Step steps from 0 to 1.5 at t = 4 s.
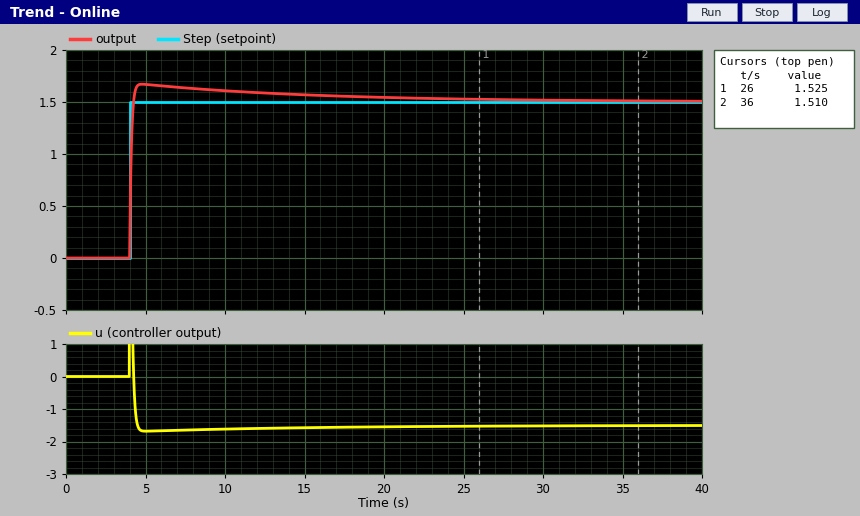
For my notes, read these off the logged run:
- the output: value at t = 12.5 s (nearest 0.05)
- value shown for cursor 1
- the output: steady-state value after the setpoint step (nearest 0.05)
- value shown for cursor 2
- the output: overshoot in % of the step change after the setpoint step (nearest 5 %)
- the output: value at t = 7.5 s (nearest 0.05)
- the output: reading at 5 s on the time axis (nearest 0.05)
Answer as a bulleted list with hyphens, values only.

- 1.60
- 1.525
- 1.50
- 1.510
- 10 %
- 1.65
- 1.65
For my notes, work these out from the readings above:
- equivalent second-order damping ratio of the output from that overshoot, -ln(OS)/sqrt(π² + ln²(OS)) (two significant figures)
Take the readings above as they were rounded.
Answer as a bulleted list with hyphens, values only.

- 0.59
